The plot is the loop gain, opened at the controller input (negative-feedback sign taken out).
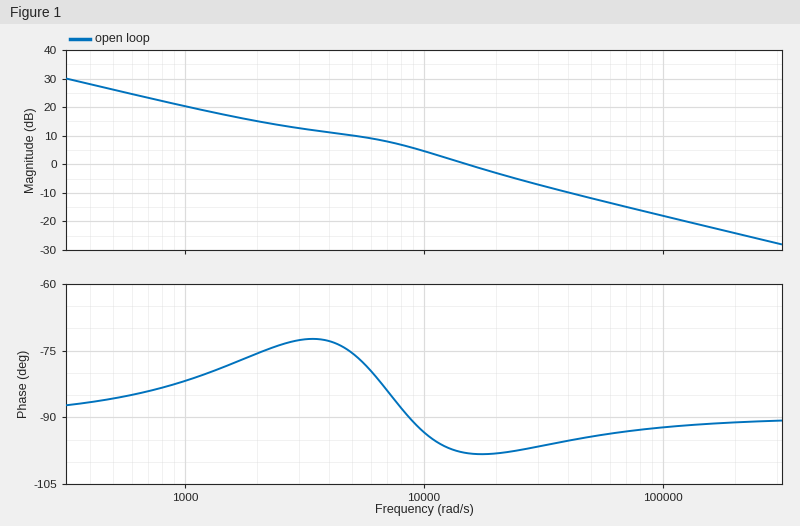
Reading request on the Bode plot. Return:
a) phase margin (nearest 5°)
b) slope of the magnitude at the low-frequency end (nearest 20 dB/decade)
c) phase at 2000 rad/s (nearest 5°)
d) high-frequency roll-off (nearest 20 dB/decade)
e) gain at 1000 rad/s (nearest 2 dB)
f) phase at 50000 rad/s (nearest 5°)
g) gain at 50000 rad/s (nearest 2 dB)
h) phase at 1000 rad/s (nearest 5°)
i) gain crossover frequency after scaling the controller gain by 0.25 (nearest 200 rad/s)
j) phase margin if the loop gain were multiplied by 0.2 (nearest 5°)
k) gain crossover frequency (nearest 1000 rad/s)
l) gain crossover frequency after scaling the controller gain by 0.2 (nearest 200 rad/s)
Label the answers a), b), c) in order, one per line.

a) 80°
b) -20 dB/decade
c) -75°
d) -20 dB/decade
e) 20 dB
f) -95°
g) -12 dB
h) -80°
i) 3400 rad/s
j) 105°
k) 15000 rad/s
l) 2400 rad/s
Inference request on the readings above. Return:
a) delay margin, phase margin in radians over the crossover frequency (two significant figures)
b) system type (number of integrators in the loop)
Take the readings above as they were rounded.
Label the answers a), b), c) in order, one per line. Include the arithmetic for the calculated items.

a) 80 × π / 180 / 15000 = 0.000093 s
b) 1
